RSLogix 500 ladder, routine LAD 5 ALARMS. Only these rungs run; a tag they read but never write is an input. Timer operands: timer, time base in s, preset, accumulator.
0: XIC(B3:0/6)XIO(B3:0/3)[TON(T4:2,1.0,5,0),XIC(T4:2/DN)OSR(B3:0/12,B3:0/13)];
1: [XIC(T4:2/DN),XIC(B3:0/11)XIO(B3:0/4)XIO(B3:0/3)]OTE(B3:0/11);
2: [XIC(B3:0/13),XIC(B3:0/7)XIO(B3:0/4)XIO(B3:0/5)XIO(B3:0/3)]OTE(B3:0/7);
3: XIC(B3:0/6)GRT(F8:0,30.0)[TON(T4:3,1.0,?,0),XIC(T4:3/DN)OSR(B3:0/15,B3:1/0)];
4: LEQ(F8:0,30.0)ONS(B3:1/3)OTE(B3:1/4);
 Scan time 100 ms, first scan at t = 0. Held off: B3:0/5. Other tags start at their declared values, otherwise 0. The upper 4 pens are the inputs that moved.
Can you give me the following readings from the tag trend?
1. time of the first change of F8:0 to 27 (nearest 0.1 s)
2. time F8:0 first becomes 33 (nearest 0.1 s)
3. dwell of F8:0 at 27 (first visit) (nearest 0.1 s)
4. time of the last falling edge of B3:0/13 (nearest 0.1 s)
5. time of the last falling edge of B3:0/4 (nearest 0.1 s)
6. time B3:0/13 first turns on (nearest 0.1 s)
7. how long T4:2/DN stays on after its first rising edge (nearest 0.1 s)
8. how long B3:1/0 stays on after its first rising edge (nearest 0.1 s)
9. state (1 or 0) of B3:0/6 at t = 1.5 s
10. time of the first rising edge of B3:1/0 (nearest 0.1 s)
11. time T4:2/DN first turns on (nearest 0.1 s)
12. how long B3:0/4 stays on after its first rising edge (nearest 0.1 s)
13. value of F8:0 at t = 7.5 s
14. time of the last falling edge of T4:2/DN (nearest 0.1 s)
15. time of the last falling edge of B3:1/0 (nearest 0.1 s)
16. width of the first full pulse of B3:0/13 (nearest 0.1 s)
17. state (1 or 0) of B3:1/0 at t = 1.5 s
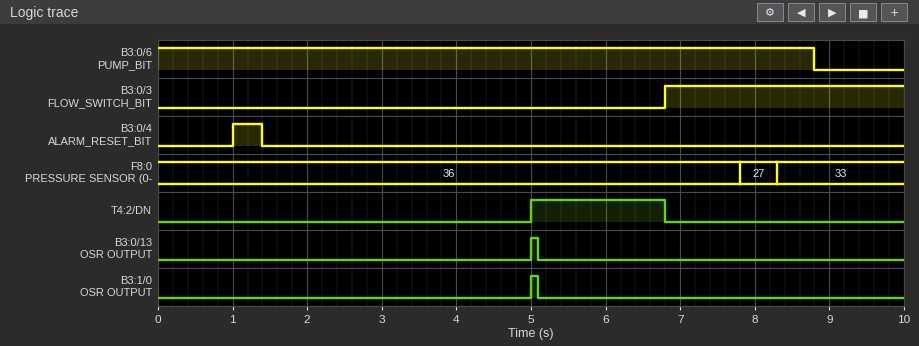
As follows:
7.8 s
8.3 s
0.5 s
5.1 s
1.4 s
5.0 s
1.8 s
0.1 s
1
5.0 s
5.0 s
0.4 s
36
6.8 s
5.1 s
0.1 s
0
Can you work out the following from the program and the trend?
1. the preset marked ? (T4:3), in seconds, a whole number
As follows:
5 s
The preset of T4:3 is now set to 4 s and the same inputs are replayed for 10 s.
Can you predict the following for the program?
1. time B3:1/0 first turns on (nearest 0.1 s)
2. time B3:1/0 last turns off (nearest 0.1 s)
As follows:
4.0 s
4.1 s
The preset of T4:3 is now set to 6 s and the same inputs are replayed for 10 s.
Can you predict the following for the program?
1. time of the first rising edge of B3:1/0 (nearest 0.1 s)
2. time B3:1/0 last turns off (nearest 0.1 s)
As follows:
6.0 s
6.1 s
